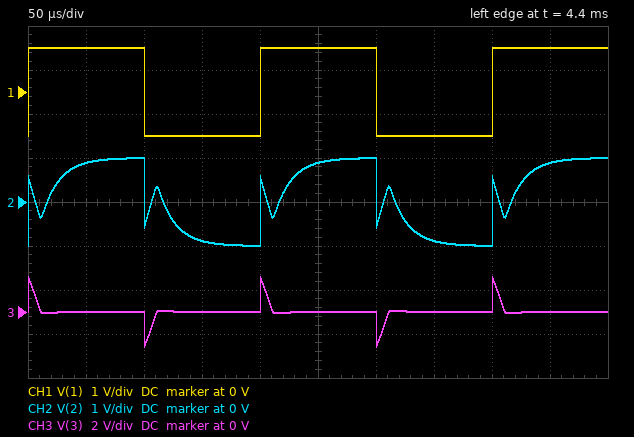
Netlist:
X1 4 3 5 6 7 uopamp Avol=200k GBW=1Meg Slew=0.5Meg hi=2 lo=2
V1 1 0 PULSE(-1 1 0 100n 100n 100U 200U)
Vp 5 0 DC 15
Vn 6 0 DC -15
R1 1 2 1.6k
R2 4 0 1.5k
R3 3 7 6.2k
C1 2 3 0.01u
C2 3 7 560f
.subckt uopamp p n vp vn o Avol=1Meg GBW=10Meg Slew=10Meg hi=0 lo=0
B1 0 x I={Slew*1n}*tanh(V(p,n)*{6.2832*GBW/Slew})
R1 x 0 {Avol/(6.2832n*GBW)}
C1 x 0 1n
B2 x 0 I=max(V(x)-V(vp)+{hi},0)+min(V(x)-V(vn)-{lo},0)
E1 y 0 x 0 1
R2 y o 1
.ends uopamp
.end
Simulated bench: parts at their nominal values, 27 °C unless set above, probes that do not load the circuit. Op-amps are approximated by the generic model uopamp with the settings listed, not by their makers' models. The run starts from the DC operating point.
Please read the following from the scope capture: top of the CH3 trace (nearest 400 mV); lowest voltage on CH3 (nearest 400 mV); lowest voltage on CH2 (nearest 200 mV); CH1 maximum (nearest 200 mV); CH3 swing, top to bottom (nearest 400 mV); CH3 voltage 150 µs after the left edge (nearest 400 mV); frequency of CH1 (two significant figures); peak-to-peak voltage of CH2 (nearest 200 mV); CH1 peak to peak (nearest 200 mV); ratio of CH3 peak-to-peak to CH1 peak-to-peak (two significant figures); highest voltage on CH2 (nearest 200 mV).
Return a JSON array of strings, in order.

["1.6 V", "-1.6 V", "-1.0 V", "1.0 V", "3.2 V", "0 V", "5.0 kHz", "2.0 V", "2.0 V", "1.6", "1.0 V"]
